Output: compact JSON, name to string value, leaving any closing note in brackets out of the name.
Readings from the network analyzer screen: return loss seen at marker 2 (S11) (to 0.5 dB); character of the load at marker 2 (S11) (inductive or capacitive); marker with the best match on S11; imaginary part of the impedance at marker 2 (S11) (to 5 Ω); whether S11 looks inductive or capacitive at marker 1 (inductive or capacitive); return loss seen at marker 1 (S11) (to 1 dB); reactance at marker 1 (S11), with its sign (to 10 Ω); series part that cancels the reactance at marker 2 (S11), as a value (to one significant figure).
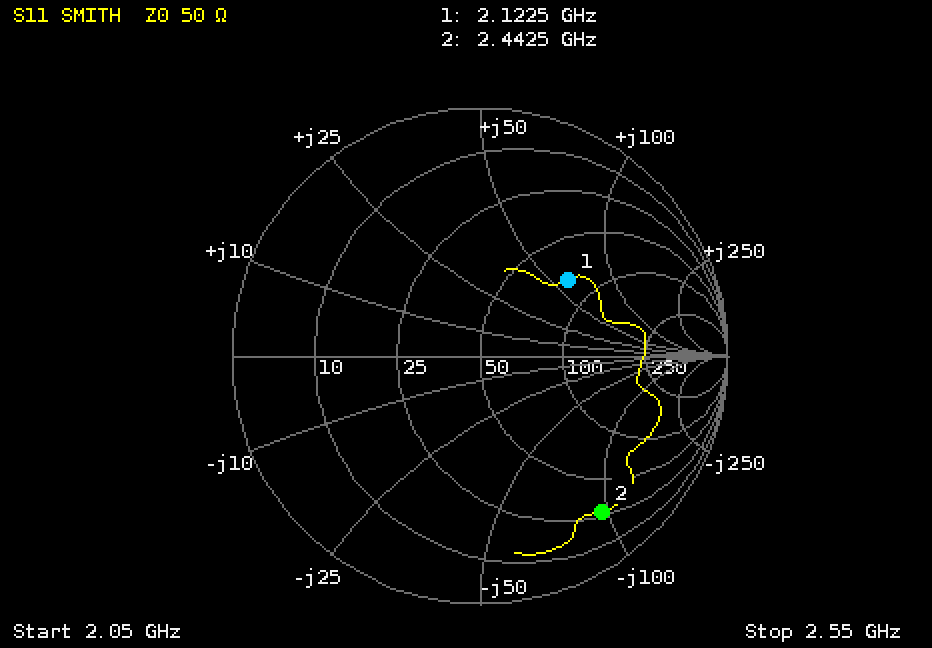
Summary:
{"return loss seen at marker 2 (S11)": "2.0 dB", "character of the load at marker 2 (S11)": "capacitive", "marker with the best match on S11": "marker 1", "imaginary part of the impedance at marker 2 (S11)": "-95 Ω", "whether S11 looks inductive or capacitive at marker 1": "inductive", "return loss seen at marker 1 (S11)": "7 dB", "reactance at marker 1 (S11), with its sign": "+60 Ω", "series part that cancels the reactance at marker 2 (S11), as a value": "6 nH"}
